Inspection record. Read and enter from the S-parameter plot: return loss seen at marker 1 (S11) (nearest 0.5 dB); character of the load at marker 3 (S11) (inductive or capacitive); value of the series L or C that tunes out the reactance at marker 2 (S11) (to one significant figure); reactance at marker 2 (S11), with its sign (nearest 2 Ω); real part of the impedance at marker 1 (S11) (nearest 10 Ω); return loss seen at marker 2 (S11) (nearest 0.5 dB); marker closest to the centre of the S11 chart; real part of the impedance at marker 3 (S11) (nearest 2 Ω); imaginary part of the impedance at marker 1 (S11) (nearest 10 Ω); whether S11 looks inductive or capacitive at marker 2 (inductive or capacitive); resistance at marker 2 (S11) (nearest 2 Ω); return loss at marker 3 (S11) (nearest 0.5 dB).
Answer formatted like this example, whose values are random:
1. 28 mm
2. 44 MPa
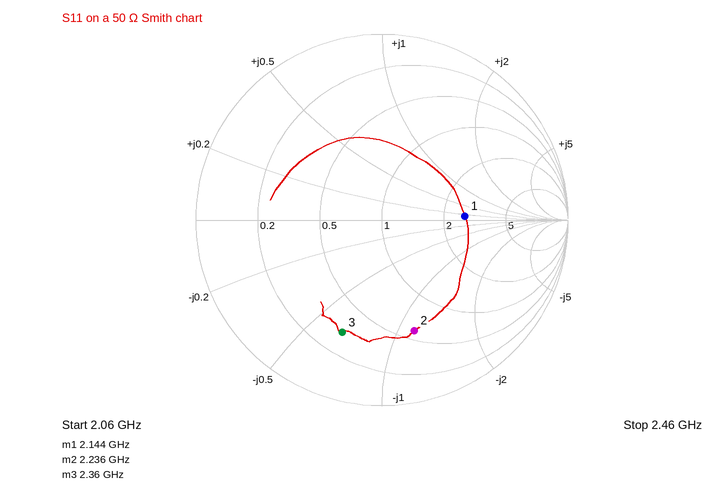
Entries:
1. 7.0 dB
2. capacitive
3. 4 nH
4. -58 Ω
5. 130 Ω
6. 4.0 dB
7. marker 1
8. 16 Ω
9. +10 Ω
10. capacitive
11. 30 Ω
12. 4.0 dB
